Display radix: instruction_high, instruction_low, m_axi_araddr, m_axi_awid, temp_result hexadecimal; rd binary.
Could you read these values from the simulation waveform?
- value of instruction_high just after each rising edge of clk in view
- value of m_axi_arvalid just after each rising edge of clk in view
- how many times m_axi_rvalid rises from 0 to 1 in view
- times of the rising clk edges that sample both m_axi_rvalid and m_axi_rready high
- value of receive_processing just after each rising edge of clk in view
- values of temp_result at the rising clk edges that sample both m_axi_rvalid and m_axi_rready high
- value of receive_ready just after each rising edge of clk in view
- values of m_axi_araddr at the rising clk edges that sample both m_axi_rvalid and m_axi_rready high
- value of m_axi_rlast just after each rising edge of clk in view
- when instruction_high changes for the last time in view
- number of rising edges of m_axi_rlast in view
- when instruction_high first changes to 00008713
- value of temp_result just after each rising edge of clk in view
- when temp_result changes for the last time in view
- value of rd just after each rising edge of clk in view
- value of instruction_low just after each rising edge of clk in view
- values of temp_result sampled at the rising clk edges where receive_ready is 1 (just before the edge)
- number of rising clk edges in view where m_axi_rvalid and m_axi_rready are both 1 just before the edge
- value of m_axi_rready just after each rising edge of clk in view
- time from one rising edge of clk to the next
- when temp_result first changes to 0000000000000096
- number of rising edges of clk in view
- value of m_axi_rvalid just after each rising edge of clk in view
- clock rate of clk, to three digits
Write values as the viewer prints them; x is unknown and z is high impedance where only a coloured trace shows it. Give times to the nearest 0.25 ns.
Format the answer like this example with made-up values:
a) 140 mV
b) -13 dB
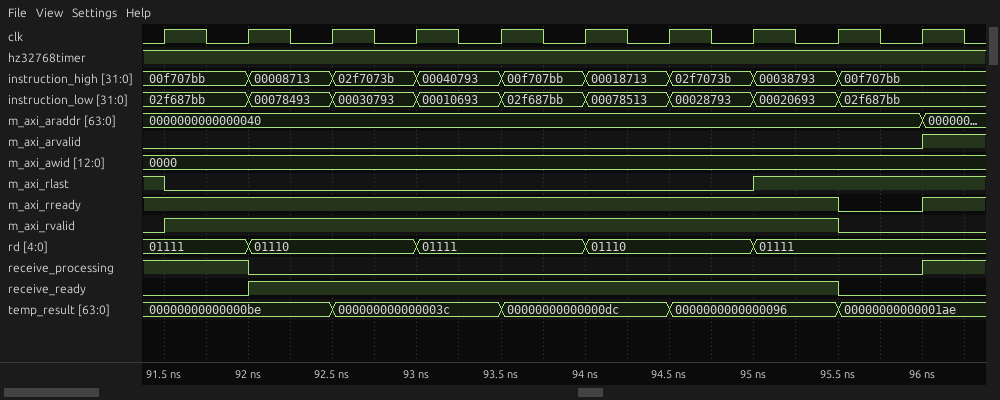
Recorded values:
a) 00f707bb, 00008713, 02f7073b, 00040793, 00f707bb, 00018713, 02f7073b, 00038793, 00f707bb, 00f707bb
b) 0 0 0 0 0 0 0 0 0 1
c) 1
d) 92 ns, 92.5 ns, 93 ns, 93.5 ns, 94 ns, 94.5 ns, 95 ns, 95.5 ns
e) 1 0 0 0 0 0 0 0 0 1
f) 00000000000000be, 00000000000000be, 000000000000003c, 000000000000003c, 00000000000000dc, 00000000000000dc, 0000000000000096, 0000000000000096
g) 0 1 1 1 1 1 1 1 0 0
h) 0000000000000040, 0000000000000040, 0000000000000040, 0000000000000040, 0000000000000040, 0000000000000040, 0000000000000040, 0000000000000040
i) 0 0 0 0 0 0 0 1 1 1
j) 95.5 ns
k) 1
l) 92 ns
m) 00000000000000be, 00000000000000be, 000000000000003c, 000000000000003c, 00000000000000dc, 00000000000000dc, 0000000000000096, 0000000000000096, 00000000000001ae, 00000000000001ae
n) 95.5 ns
o) 01111, 01110, 01110, 01111, 01111, 01110, 01110, 01111, 01111, 01111
p) 02f687bb, 00078493, 00030793, 00010693, 02f687bb, 00078513, 00028793, 00020693, 02f687bb, 02f687bb
q) 00000000000000be, 000000000000003c, 000000000000003c, 00000000000000dc, 00000000000000dc, 0000000000000096, 0000000000000096
r) 8
s) 1 1 1 1 1 1 1 1 0 1
t) 0.5 ns
u) 94.5 ns
v) 10
w) 1 1 1 1 1 1 1 1 0 0
x) 2.00 GHz
